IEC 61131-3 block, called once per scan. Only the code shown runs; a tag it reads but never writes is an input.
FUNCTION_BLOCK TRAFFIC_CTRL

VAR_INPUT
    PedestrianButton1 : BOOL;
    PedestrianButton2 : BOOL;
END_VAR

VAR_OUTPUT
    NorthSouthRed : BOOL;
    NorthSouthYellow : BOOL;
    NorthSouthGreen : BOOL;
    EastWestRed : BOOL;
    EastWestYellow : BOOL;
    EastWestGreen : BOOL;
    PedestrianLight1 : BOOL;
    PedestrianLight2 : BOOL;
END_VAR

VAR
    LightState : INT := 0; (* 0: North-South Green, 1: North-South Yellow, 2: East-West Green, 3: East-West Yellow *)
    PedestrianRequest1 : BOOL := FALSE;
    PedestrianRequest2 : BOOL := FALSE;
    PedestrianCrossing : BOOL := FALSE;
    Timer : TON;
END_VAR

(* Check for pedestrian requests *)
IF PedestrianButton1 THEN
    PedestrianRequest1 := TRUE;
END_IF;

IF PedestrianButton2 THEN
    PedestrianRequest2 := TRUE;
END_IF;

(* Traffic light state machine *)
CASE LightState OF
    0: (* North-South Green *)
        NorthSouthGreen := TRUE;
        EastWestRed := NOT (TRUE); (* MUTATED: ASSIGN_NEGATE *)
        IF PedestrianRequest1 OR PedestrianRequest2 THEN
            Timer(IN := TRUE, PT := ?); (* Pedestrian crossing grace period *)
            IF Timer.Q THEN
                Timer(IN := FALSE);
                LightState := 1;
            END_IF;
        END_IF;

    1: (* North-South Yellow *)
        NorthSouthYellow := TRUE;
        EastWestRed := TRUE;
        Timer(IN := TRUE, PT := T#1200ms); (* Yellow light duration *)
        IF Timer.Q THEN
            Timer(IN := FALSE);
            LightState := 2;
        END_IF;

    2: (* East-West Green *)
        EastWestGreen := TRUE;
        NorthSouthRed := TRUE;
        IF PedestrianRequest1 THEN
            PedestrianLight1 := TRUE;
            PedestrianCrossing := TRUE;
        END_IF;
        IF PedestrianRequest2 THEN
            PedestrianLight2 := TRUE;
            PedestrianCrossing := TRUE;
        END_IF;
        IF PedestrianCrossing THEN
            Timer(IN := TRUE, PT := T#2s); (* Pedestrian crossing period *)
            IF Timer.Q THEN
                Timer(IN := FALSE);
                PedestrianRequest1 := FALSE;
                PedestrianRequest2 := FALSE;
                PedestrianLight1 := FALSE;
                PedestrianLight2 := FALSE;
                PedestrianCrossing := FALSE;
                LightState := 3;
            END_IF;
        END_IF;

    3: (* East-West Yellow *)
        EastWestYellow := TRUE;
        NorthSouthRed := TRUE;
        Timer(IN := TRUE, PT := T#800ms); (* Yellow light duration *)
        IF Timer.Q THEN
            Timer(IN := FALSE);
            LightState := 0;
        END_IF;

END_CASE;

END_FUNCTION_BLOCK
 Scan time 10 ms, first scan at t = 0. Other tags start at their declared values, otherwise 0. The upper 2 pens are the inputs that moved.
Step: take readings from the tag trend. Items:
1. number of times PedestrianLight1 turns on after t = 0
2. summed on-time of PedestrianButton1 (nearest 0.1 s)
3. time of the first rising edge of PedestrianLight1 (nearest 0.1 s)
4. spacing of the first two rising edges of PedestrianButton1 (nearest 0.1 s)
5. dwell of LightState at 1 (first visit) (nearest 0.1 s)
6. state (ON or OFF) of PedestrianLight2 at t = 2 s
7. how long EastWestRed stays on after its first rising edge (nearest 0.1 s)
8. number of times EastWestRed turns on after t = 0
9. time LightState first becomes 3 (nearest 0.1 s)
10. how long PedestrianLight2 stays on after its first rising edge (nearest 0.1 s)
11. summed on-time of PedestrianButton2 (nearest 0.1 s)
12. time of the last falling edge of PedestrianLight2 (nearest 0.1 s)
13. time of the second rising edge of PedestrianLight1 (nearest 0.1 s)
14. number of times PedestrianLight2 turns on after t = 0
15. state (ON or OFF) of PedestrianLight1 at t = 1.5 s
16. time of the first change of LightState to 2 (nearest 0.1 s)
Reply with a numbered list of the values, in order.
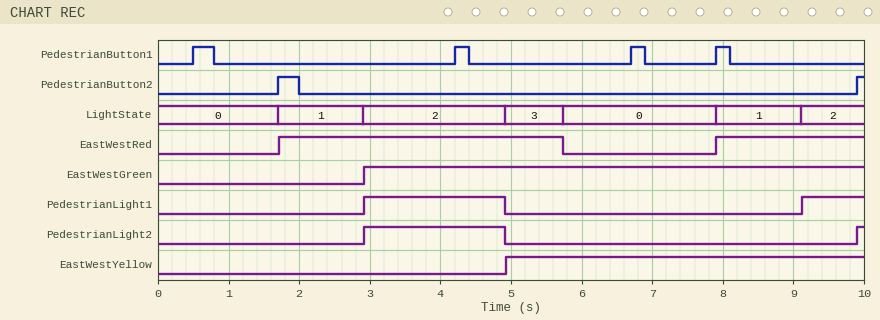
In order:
1. 2
2. 0.9 s
3. 2.9 s
4. 3.7 s
5. 1.2 s
6. OFF
7. 4.0 s
8. 2
9. 4.9 s
10. 2.0 s
11. 0.4 s
12. 4.9 s
13. 9.1 s
14. 2
15. OFF
16. 2.9 s
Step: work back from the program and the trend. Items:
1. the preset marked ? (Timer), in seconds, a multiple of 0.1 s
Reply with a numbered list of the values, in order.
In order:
1. 1.2 s
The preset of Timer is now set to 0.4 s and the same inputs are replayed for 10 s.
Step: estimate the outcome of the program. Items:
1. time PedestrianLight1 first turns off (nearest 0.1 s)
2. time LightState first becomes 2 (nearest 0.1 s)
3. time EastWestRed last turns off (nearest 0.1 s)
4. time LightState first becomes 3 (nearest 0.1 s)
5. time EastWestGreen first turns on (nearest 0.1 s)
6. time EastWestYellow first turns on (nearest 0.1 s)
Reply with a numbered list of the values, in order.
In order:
1. 4.1 s
2. 2.1 s
3. 9.4 s
4. 4.1 s
5. 2.1 s
6. 4.1 s
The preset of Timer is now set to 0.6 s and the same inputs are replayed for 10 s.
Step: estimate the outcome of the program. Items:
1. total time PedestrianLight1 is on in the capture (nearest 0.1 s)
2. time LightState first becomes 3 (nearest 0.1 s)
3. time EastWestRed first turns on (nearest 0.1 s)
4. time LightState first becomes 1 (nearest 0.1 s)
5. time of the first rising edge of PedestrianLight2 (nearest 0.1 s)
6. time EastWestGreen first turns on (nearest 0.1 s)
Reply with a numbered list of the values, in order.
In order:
1. 4.0 s
2. 4.3 s
3. 1.1 s
4. 1.1 s
5. 2.3 s
6. 2.3 s
